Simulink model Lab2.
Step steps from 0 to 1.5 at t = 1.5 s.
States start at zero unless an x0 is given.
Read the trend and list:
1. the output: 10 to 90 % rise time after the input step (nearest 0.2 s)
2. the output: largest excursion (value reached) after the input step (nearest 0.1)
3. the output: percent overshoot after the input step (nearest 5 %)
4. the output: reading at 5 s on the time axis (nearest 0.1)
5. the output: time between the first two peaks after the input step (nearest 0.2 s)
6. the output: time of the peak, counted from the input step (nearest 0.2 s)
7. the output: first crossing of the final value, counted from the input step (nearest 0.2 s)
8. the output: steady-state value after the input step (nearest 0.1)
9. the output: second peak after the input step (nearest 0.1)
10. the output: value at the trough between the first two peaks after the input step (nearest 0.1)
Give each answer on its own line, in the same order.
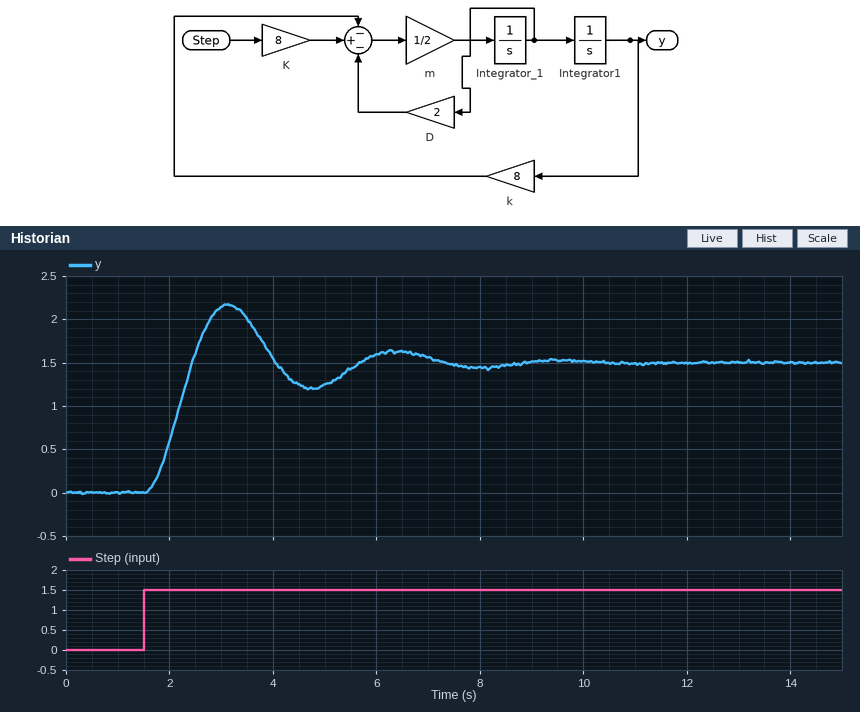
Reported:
0.6 s
2.2
45 %
1.2
3.2 s
1.6 s
1.0 s
1.5
1.6
1.2
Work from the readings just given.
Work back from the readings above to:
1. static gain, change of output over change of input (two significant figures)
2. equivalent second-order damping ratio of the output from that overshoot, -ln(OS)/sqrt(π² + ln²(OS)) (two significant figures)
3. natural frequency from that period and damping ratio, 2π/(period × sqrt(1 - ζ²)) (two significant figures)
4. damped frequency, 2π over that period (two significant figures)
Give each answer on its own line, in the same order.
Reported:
1.0
0.25
2.0 rad/s
2.0 rad/s
